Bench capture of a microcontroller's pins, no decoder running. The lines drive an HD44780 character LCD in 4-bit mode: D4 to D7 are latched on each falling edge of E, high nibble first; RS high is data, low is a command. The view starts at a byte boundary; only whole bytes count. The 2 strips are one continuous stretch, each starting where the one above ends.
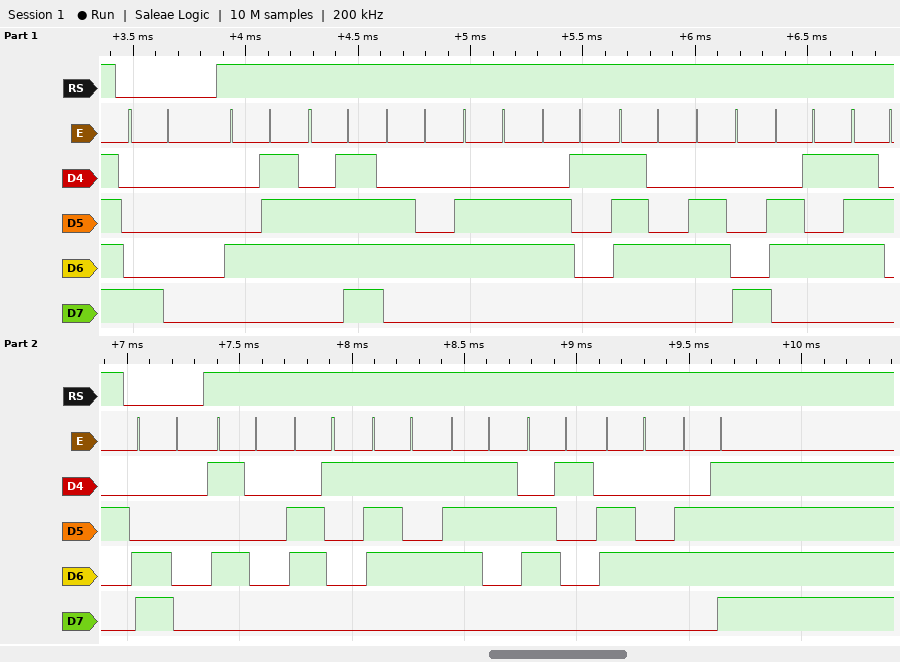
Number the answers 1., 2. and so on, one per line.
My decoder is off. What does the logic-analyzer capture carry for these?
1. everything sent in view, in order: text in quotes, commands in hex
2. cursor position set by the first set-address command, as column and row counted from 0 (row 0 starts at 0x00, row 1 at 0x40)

1. 0x80 "Godfather" 0xC0 "Pausado"
2. column 0, row 0
